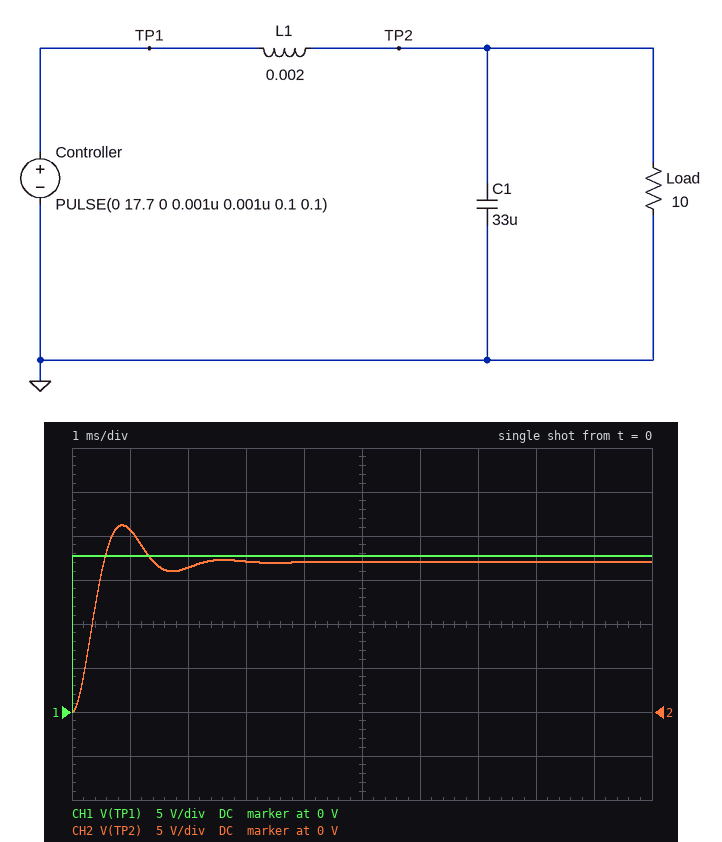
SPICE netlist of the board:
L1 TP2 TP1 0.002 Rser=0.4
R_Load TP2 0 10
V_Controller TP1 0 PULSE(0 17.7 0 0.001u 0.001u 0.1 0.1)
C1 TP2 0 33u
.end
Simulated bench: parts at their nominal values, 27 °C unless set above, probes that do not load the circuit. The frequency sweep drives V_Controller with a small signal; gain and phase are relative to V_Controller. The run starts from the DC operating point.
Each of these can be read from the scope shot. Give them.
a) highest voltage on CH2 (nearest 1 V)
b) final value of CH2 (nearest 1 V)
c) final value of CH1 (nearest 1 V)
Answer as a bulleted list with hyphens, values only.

- 21 V
- 17 V
- 18 V
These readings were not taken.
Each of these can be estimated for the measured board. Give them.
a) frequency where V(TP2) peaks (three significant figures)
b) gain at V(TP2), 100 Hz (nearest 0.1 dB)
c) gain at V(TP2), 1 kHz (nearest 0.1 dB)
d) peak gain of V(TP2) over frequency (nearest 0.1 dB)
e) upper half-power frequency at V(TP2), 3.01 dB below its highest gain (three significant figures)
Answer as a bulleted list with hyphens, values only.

- 517 Hz
- -0.2 dB
- -6.3 dB
- 2.2 dB
- 751 Hz
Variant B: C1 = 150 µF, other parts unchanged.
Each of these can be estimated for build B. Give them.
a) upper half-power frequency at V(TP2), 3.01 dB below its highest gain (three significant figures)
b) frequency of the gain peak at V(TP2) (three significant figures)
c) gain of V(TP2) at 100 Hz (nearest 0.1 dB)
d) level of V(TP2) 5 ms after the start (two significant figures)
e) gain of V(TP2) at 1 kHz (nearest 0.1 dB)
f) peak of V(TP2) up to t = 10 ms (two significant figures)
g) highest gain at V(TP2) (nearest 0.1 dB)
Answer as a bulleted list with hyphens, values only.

- 344 Hz
- 280 Hz
- 0.6 dB
- 19 V
- -20.8 dB
- 25 V
- 6.5 dB
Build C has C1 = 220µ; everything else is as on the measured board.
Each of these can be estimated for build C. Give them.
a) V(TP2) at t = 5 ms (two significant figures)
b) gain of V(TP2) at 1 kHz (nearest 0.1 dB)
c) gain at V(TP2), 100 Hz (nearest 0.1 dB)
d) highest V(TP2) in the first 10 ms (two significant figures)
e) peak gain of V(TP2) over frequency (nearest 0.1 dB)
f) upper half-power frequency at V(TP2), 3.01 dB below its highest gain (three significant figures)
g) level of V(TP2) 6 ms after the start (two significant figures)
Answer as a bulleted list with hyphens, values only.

- 15 V
- -24.3 dB
- 1.1 dB
- 26 V
- 7.3 dB
- 282 Hz
- 19 V
